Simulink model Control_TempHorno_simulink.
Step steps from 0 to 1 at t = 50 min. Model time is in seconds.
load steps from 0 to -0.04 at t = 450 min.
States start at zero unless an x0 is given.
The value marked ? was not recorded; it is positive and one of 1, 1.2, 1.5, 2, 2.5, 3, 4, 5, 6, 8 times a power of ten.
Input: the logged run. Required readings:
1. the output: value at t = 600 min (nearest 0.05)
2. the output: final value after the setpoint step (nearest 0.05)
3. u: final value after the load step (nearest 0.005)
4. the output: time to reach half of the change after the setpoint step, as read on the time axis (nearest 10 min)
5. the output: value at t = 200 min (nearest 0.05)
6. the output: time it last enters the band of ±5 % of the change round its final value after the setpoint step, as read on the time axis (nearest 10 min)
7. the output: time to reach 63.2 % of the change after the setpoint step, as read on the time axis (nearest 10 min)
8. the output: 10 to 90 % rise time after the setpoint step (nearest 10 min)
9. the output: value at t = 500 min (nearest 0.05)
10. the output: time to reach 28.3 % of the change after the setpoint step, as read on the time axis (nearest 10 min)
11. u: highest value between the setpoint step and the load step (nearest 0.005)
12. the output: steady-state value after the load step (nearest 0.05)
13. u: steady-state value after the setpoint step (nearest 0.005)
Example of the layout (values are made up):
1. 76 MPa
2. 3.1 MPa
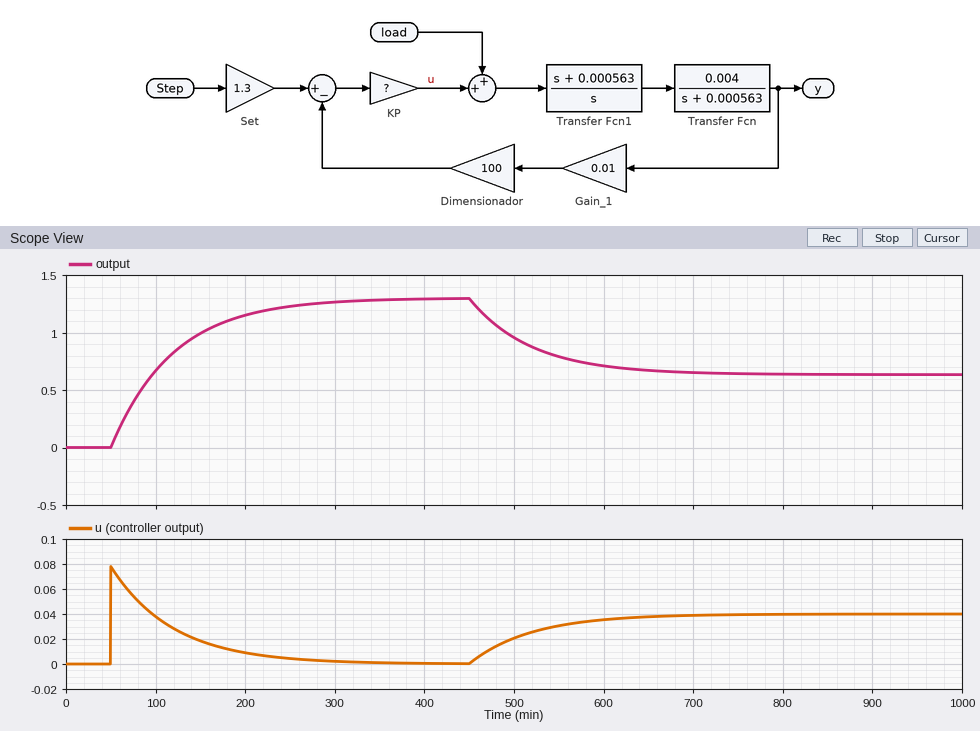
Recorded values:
1. 0.70
2. 1.30
3. 0.040
4. 100 min
5. 1.15
6. 260 min
7. 120 min
8. 150 min
9. 0.95
10. 70 min
11. 0.080
12. 0.65
13. 0.000
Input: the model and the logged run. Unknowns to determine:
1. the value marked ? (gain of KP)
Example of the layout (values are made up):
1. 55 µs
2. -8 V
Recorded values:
1. 0.06
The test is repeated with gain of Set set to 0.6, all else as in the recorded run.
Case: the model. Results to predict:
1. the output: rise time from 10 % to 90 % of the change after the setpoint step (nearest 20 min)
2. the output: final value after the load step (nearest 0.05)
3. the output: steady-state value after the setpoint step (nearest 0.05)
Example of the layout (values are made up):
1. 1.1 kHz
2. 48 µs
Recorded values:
1. 160 min
2. -0.05
3. 0.60
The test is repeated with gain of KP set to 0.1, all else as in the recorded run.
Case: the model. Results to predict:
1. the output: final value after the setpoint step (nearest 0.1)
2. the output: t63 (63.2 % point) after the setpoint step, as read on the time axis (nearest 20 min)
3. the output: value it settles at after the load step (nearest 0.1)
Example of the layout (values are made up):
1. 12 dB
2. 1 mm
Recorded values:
1. 1.3
2. 100 min
3. 0.9
